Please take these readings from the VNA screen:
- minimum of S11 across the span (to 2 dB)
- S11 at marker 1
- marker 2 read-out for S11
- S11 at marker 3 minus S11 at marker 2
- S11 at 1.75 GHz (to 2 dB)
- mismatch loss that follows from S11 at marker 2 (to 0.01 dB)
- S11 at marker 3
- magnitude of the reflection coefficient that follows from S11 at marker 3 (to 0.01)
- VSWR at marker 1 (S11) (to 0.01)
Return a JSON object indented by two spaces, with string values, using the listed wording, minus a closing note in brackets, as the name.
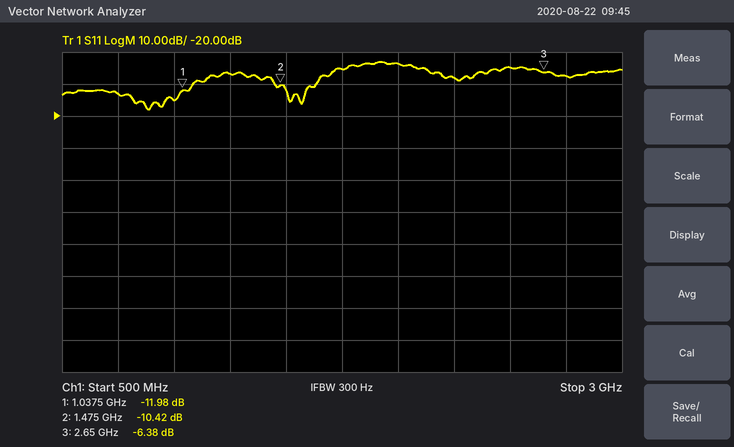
{
  "minimum of S11 across the span": "-18 dB",
  "S11 at marker 1": "-11.98 dB",
  "marker 2 read-out for S11": "-10.42 dB",
  "S11 at marker 3 minus S11 at marker 2": "4.04 dB",
  "S11 at 1.75 GHz": "-6 dB",
  "mismatch loss that follows from S11 at marker 2": "0.41 dB",
  "S11 at marker 3": "-6.38 dB",
  "magnitude of the reflection coefficient that follows from S11 at marker 3": "0.48",
  "VSWR at marker 1 (S11)": "1.67"
}
